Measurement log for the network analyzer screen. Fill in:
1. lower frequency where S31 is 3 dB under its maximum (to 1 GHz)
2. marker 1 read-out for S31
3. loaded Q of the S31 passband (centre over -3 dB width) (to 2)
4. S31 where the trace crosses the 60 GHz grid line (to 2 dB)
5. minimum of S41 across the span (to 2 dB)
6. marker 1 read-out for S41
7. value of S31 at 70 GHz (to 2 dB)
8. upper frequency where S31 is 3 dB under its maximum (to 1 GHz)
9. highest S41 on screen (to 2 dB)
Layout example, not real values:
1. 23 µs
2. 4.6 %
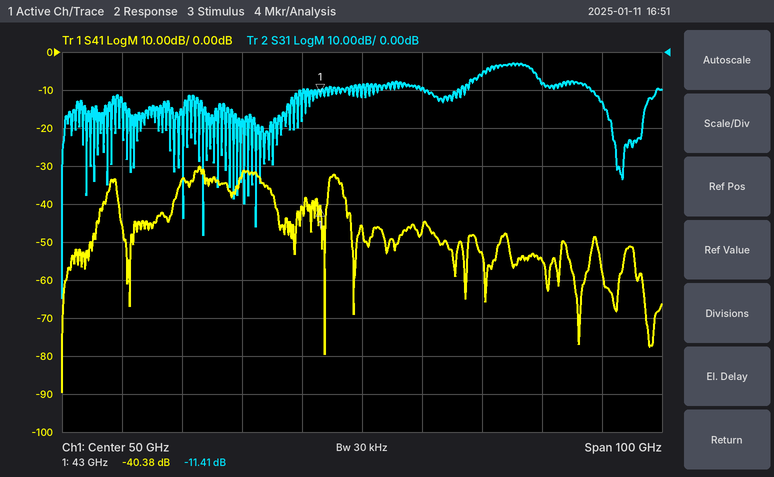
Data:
1. 70 GHz
2. -11.41 dB
3. 8
4. -10 dB
5. -90 dB
6. -40.38 dB
7. -6 dB
8. 79 GHz
9. -30 dB
